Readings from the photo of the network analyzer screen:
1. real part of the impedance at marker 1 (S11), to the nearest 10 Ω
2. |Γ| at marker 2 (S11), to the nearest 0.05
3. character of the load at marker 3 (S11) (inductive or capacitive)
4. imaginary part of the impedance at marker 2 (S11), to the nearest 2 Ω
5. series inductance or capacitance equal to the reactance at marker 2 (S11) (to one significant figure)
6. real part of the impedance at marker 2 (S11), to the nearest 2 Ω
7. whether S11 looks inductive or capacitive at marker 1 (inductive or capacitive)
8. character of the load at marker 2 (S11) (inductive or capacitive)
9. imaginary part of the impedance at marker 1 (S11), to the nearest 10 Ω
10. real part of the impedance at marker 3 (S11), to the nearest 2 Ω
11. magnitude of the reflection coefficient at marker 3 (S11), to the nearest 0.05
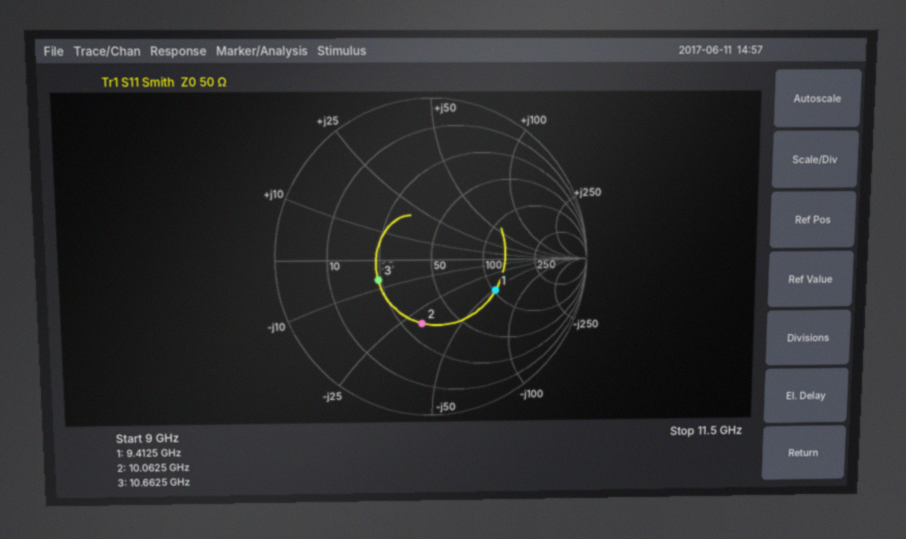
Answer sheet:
100 Ω
0.40
capacitive
-32 Ω
500 fF
32 Ω
capacitive
capacitive
-50 Ω
24 Ω
0.35
